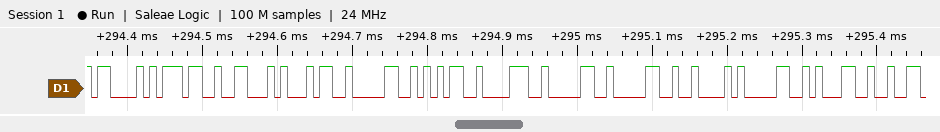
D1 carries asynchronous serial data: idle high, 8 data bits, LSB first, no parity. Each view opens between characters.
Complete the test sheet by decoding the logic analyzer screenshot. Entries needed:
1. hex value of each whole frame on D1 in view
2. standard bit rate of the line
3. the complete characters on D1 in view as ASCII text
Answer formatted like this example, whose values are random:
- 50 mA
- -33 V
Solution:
- 43, 37, 46, 34, 30, 35, 38, 30, 30, 42, 30, 31
- 115200 baud
- "C7F405800B01"
